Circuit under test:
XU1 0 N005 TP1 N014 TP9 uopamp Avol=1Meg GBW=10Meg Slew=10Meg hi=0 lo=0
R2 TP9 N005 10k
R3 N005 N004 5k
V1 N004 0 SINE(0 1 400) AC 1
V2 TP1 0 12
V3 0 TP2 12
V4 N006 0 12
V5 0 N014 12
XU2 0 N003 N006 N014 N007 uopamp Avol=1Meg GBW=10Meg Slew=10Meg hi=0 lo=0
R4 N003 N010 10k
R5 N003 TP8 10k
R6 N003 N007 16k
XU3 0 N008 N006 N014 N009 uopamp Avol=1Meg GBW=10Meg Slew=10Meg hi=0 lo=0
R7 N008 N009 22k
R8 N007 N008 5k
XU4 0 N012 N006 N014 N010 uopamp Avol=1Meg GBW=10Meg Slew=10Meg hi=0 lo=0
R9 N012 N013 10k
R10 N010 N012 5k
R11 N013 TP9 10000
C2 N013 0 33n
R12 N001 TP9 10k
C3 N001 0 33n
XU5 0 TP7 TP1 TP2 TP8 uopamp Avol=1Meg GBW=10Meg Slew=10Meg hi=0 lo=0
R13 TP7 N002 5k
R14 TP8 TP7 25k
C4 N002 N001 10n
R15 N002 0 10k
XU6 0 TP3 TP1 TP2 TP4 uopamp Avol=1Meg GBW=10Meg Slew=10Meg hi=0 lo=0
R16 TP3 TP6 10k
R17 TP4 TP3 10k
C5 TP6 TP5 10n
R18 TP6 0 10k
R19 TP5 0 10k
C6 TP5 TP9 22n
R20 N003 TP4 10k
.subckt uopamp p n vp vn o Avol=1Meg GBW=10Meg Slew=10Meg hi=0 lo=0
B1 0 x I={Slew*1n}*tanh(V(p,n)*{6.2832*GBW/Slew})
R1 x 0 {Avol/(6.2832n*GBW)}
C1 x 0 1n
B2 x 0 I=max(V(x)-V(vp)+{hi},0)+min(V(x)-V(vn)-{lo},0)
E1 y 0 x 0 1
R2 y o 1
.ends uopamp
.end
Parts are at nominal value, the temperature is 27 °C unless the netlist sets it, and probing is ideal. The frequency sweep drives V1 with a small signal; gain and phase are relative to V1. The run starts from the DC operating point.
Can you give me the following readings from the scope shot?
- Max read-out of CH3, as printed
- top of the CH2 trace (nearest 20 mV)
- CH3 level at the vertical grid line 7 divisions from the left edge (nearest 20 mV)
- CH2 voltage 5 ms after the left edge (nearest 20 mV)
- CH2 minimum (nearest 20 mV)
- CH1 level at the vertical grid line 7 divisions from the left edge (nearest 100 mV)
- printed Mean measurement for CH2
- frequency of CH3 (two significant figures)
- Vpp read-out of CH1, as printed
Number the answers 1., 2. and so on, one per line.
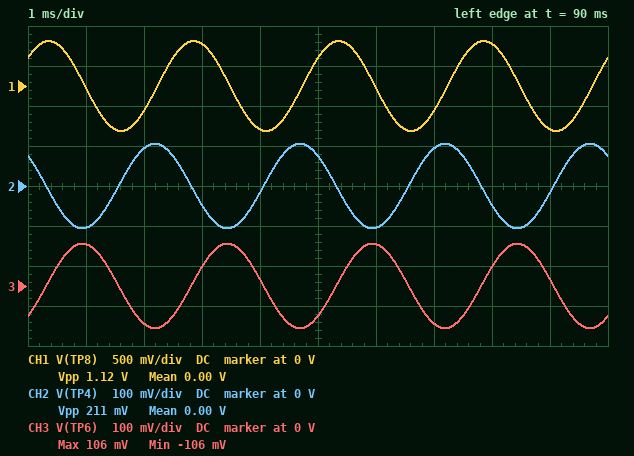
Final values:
1. 106 mV
2. 100 mV
3. -100 mV
4. 80 mV
5. -100 mV
6. -300 mV
7. 0.00 V
8. 400 Hz
9. 1.12 V
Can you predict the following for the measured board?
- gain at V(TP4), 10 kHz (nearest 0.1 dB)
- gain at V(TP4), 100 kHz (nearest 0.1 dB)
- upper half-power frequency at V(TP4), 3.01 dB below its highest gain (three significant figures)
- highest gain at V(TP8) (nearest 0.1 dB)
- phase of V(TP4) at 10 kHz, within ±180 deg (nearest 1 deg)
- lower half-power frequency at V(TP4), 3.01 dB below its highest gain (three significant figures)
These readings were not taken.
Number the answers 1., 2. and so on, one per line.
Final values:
1. 5.1 dB
2. 6.0 dB
3. 2.56 MHz
4. -2.9 dB
5. 28 deg
6. 4.91 kHz
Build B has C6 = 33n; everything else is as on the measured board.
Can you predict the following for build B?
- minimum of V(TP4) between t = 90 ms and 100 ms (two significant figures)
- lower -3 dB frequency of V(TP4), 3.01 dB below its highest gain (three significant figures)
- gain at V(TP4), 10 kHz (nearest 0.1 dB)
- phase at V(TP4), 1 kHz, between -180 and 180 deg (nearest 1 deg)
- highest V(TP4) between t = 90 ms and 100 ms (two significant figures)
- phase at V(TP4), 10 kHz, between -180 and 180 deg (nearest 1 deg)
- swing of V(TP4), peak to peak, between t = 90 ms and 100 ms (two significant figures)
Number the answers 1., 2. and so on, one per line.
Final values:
1. -140 mV
2. 4.29 kHz
3. 5.3 dB
4. 97 deg
5. 140 mV
6. 25 deg
7. 280 mV
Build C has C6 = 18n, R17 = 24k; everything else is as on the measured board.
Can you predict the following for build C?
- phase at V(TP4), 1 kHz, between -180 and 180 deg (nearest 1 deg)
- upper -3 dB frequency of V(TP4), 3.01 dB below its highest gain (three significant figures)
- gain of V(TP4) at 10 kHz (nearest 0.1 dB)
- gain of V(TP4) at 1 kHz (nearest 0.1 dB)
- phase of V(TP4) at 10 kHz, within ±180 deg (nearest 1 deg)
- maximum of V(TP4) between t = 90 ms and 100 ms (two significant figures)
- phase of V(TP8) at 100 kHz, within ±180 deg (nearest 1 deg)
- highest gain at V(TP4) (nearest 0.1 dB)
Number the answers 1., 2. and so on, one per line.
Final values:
1. 107 deg
2. 2.02 MHz
3. 12.5 dB
4. -2.1 dB
5. 31 deg
6. 220 mV
7. -91 deg
8. 13.6 dB
